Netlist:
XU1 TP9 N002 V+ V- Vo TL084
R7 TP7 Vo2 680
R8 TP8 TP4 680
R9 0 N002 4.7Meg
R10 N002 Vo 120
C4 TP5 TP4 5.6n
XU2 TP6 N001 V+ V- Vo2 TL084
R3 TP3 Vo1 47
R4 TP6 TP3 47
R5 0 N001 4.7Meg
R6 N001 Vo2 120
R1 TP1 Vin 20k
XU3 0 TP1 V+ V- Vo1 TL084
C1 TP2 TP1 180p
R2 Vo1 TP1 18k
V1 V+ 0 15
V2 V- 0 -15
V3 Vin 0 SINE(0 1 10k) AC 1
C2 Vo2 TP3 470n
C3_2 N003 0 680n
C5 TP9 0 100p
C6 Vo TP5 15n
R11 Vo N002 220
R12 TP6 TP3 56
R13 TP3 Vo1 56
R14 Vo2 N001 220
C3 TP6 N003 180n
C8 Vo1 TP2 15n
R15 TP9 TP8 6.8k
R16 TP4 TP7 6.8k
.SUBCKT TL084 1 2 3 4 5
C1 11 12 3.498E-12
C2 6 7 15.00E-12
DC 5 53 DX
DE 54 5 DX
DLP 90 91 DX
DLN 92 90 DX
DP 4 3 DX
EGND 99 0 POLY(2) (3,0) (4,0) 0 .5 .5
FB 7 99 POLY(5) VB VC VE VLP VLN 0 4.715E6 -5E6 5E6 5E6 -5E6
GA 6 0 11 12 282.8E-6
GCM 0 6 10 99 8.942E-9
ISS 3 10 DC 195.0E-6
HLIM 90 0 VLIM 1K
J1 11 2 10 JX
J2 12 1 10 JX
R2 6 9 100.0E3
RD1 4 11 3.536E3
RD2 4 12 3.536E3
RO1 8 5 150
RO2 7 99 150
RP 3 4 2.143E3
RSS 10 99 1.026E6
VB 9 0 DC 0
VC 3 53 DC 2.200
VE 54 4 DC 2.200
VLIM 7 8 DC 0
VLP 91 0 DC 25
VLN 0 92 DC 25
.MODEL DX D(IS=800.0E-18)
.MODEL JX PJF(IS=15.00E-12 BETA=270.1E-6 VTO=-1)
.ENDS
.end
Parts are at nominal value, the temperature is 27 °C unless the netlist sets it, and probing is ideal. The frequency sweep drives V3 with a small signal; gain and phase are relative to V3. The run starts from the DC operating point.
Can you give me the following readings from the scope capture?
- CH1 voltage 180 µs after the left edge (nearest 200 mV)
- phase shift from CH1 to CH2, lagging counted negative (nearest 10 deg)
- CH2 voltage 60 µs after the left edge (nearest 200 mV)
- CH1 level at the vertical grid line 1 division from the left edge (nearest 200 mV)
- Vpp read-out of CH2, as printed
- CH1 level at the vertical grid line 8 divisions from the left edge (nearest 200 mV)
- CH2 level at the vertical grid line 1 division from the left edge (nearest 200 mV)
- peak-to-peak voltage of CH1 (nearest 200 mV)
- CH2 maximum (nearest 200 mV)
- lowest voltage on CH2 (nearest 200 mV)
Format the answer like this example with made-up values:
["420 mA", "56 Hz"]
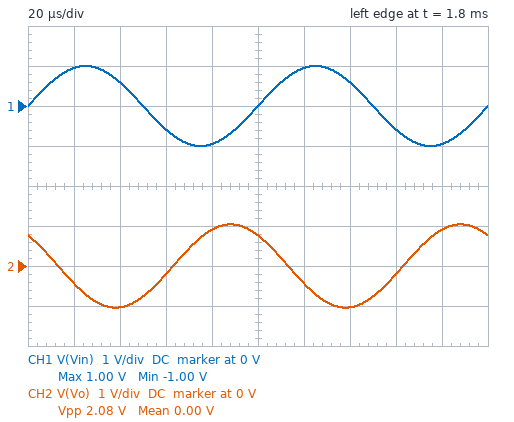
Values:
["-1.0 V", "130 deg", "-200 mV", "1.0 V", "2.08 V", "-600 mV", "-400 mV", "2.0 V", "1.0 V", "-1.0 V"]
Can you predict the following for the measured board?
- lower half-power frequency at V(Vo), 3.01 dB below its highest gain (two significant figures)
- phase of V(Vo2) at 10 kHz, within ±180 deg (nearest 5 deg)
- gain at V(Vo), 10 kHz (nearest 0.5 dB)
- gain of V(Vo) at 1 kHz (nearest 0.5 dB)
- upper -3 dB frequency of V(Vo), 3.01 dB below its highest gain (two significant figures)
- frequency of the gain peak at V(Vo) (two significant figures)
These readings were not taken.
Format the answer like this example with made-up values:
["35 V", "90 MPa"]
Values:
["14 kHz", "140 deg", "0.5 dB", "-1.0 dB", "34 kHz", "29 kHz"]
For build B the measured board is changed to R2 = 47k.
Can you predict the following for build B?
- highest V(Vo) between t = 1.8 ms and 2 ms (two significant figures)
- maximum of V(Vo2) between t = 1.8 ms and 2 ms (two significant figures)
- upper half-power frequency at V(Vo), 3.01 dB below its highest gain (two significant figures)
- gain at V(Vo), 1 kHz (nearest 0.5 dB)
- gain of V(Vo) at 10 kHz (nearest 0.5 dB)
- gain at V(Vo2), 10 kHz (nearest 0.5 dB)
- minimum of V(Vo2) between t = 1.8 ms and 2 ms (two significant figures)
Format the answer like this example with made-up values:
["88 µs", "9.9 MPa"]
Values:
["2.5 V", "2.2 V", "33 kHz", "7.5 dB", "8.0 dB", "7.0 dB", "-2.2 V"]
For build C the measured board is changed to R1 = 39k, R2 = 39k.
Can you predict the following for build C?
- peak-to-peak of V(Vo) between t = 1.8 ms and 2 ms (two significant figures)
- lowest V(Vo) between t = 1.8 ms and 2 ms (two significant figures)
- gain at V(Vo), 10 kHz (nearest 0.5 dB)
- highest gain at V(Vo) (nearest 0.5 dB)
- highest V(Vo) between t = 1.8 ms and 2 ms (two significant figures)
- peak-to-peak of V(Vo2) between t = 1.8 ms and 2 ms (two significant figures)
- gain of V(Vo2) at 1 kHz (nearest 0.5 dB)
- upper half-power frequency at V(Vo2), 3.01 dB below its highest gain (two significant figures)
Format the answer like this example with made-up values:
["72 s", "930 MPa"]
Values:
["2.2 V", "-1.1 V", "0.5 dB", "2.5 dB", "1.1 V", "2.0 V", "0 dB", "23 kHz"]
